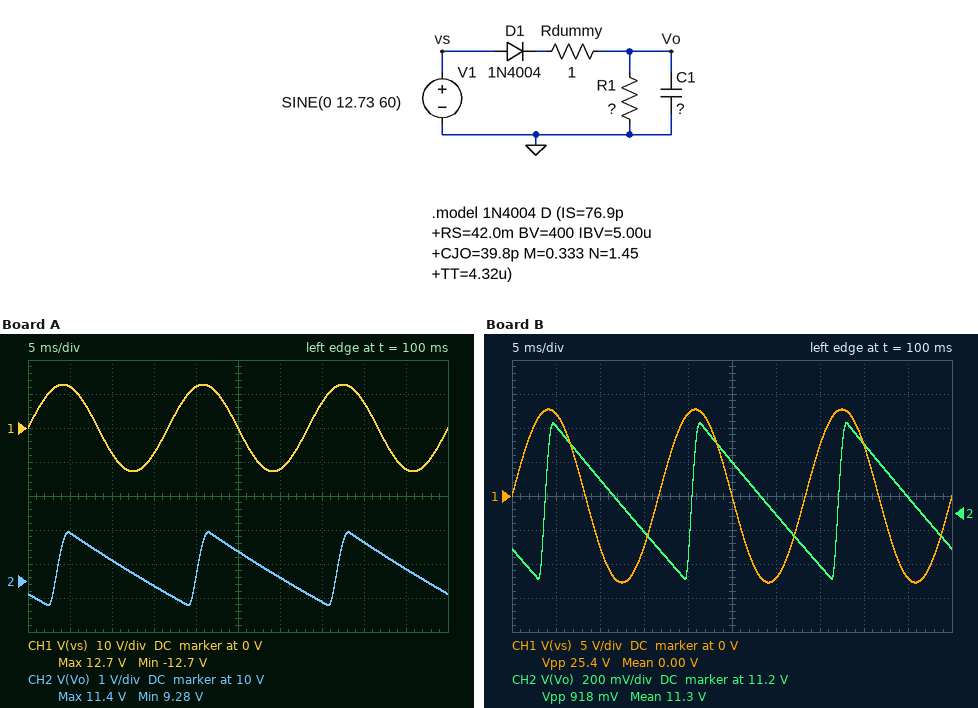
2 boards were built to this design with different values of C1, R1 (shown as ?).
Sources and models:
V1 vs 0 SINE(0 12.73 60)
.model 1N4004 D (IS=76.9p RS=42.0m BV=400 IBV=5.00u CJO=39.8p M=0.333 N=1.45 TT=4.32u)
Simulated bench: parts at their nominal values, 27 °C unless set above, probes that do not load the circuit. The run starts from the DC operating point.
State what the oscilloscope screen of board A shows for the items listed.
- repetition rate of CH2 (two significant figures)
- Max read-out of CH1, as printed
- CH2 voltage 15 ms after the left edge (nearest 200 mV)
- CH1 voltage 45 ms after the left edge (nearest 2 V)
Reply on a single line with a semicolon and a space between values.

60 Hz; 12.7 V; 9.8 V; -12 V
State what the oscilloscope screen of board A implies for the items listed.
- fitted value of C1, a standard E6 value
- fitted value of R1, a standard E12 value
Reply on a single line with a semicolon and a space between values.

680 µF; 100 Ω
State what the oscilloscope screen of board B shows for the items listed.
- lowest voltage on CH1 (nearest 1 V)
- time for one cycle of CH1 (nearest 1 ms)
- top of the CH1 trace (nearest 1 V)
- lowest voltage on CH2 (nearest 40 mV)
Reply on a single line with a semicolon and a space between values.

-13 V; 17 ms; 13 V; 10.80 V
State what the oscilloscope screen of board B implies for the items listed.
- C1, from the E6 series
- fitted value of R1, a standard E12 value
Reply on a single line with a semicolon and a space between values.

470 µF; 390 Ω
